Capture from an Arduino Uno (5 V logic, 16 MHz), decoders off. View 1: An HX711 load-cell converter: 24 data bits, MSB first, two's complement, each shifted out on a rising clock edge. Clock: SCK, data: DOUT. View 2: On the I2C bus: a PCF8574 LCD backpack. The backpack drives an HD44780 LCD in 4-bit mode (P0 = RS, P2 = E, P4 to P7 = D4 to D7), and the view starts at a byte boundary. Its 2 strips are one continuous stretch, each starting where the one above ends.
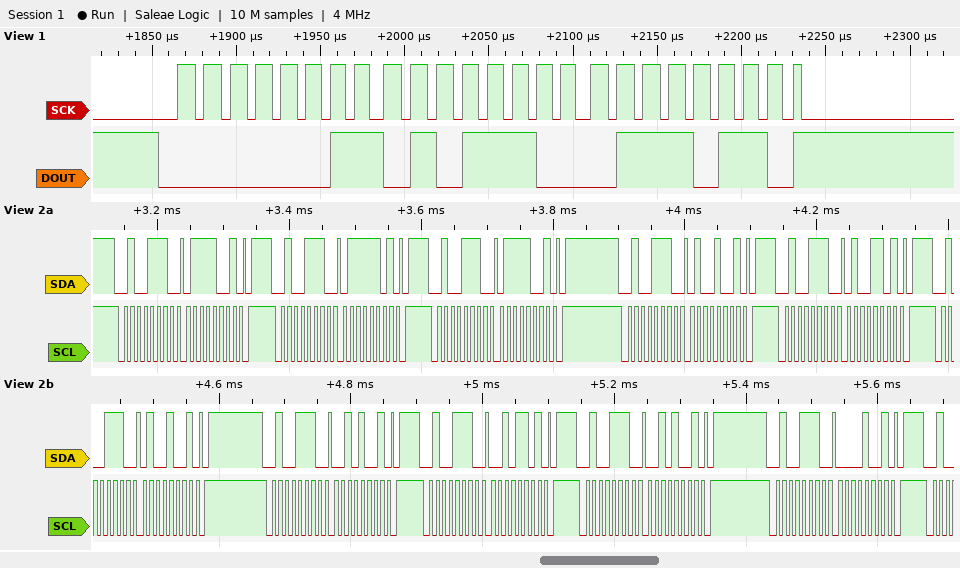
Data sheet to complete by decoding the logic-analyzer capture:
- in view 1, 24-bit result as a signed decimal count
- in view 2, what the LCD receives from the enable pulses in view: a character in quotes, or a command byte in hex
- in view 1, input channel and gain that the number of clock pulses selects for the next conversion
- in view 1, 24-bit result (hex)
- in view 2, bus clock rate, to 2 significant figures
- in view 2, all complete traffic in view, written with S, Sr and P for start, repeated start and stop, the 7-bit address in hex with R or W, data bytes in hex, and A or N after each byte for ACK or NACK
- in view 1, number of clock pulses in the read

220278
't'
channel A, gain 128
0x035C76
100 kHz
S 27W A 79 A P S 27W A 7D A P S 27W A 79 A P S 27W A 49 A P S 27W A 4D A P S 27W A 49 A P S 27W A 29 A P S 27W A 2D A P S 27W A 29 A P S 27W A 09 A P
25
